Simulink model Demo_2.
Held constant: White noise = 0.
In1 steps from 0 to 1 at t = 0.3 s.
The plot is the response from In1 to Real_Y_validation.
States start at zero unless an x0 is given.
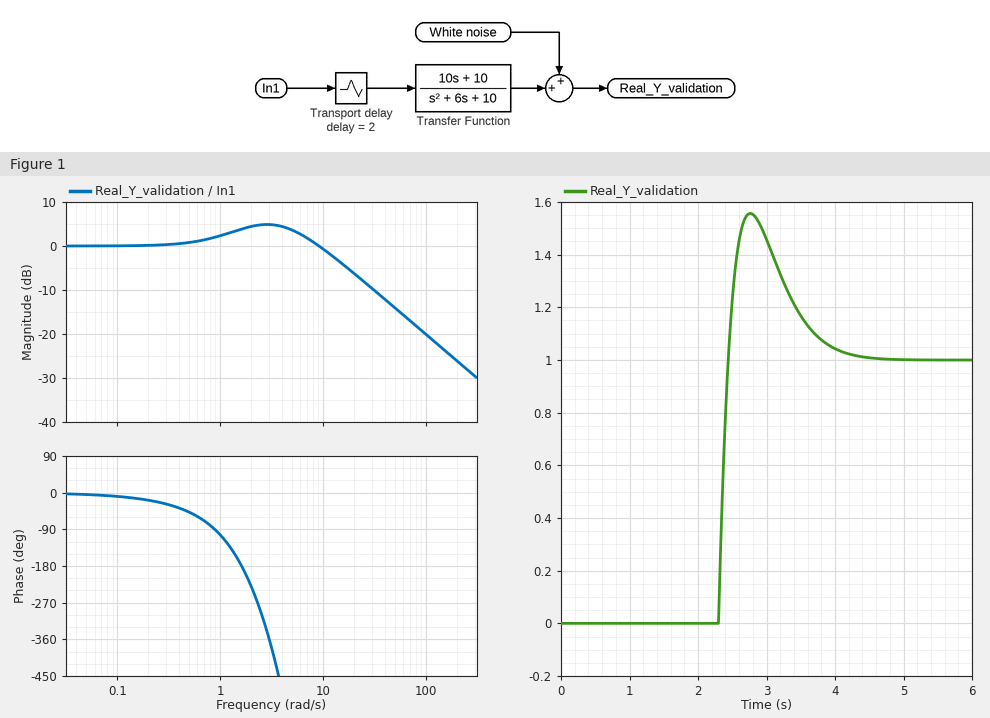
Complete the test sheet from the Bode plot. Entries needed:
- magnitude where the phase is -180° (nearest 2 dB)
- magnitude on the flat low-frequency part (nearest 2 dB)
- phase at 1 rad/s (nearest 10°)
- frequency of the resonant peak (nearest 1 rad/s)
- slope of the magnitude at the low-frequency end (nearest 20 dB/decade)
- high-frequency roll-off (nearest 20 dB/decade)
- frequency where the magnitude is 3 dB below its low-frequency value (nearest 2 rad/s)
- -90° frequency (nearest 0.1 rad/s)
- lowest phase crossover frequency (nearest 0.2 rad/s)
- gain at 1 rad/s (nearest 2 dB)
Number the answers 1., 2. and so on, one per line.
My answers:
1. 4 dB
2. 0 dB
3. -100°
4. 3 rad/s
5. 0 dB/decade
6. -20 dB/decade
7. 14 rad/s
8. 0.9 rad/s
9. 1.6 rad/s
10. 2 dB
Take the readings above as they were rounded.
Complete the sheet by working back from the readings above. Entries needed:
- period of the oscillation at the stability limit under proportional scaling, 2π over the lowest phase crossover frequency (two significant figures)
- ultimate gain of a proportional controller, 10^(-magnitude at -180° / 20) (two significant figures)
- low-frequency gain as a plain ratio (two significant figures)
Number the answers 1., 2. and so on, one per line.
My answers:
1. 3.9 s
2. 0.63
3. 1.0
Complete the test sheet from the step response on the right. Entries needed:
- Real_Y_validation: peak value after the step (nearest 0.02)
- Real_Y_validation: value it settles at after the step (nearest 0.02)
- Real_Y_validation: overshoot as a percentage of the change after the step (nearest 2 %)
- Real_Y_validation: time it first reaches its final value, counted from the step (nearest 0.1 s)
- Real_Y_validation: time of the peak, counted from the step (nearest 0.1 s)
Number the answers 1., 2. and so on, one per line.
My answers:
1. 1.56
2. 1.00
3. 56 %
4. 2.1 s
5. 2.5 s
